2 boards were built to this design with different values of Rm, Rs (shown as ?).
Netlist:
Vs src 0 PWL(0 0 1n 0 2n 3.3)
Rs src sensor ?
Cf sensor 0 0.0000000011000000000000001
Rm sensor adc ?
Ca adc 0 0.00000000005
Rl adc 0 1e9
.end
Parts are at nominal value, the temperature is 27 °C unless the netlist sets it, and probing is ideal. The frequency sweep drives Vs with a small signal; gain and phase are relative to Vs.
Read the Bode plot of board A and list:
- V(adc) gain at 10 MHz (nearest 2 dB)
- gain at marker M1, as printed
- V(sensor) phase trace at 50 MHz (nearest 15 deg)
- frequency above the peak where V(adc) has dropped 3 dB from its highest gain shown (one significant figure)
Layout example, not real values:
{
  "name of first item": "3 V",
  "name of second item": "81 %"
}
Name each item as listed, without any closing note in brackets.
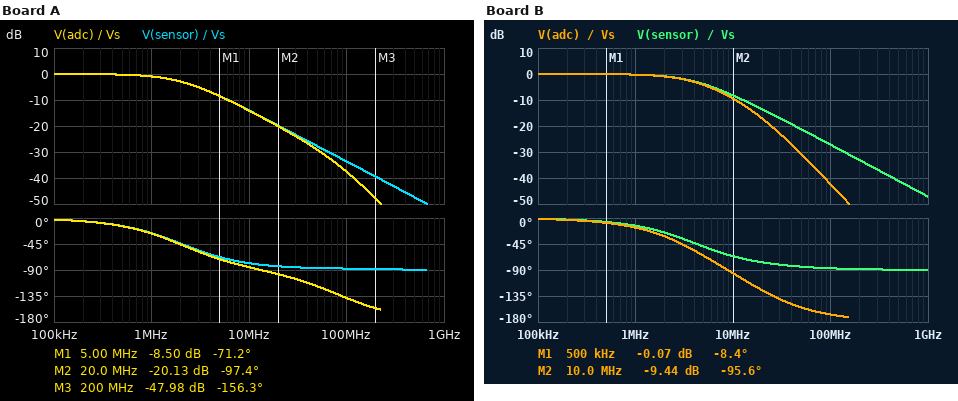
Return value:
{
  "V(adc) gain at 10 MHz": "-14 dB",
  "gain at marker M1, as printed": "-8.50 dB",
  "V(sensor) phase trace at 50 MHz": "-90 deg",
  "frequency above the peak where V(adc) has dropped 3 dB from its highest gain shown": "2 MHz"
}
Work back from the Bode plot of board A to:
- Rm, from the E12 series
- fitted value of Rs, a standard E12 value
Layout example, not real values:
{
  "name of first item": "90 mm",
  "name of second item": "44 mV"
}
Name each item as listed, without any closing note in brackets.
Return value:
{
  "Rm, from the E12 series": "39 Ω",
  "fitted value of Rs, a standard E12 value": "68 Ω"
}
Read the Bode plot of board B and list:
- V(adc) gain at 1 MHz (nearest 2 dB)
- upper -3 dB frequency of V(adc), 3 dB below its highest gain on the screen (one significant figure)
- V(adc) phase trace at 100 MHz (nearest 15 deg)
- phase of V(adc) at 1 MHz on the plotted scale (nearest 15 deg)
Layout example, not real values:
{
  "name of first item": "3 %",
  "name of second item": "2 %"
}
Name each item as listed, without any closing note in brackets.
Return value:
{
  "V(adc) gain at 1 MHz": "0 dB",
  "upper -3 dB frequency of V(adc), 3 dB below its highest gain on the screen": "4 MHz",
  "V(adc) phase trace at 100 MHz": "-165 deg",
  "phase of V(adc) at 1 MHz on the plotted scale": "-15 deg"
}
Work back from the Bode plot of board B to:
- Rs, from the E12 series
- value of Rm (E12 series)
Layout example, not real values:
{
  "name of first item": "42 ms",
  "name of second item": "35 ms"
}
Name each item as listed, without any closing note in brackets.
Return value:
{
  "Rs, from the E12 series": "33 Ω",
  "value of Rm": "180 Ω"
}
